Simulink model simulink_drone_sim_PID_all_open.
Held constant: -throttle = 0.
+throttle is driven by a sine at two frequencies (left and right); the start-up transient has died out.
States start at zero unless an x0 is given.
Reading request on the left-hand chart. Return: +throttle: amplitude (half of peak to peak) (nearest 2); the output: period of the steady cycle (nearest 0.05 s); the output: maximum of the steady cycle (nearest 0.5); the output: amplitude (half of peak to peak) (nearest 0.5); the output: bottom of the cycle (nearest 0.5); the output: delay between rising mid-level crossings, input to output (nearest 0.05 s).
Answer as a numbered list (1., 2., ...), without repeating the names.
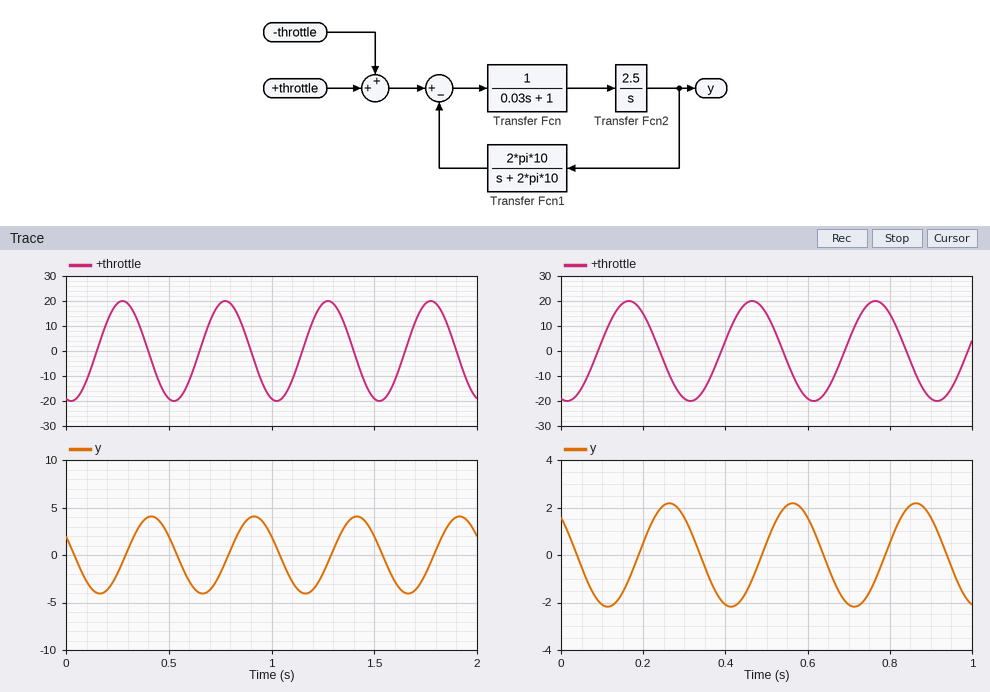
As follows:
1. 20
2. 0.50 s
3. 4.0
4. 4.0
5. -4.0
6. 0.15 s
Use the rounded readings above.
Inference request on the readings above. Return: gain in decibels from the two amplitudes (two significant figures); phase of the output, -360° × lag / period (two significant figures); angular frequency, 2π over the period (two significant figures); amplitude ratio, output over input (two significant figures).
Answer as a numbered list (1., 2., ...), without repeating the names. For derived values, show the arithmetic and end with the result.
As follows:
1. 20 log10(4 / 20) = -14 dB
2. -360 × 0.15 / 0.5 = -110°
3. 2π / 0.5 = 13 rad/s
4. 4 / 20 = 0.20
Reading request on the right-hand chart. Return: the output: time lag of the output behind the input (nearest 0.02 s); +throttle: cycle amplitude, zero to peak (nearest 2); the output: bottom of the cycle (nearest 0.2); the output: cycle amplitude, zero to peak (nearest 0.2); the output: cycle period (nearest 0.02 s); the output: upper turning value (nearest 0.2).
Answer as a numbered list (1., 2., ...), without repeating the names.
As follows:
1. 0.10 s
2. 20
3. -2.2
4. 2.2
5. 0.30 s
6. 2.2
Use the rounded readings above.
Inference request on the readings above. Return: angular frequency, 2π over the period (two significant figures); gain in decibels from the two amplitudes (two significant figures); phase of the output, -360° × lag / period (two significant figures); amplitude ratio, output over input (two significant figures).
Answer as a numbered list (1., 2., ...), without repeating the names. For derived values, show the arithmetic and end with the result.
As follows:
1. 2π / 0.3 = 21 rad/s
2. 20 log10(2.2 / 20) = -19 dB
3. -360 × 0.1 / 0.3 = -120°
4. 2.2 / 20 = 0.11
